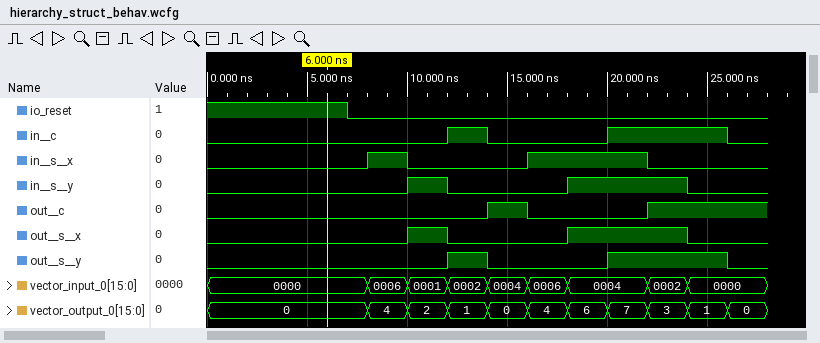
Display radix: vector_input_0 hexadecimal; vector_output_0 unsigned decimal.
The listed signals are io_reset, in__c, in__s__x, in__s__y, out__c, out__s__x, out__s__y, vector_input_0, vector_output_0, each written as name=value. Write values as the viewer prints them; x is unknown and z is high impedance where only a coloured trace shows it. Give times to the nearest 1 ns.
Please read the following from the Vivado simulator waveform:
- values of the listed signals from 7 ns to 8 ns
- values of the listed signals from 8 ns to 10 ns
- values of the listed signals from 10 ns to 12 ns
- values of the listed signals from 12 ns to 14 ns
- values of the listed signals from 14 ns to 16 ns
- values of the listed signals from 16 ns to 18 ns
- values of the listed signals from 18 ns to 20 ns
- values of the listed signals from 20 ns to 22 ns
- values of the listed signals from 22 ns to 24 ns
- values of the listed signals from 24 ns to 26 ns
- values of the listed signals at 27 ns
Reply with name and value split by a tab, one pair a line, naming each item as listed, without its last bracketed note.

values of the listed signals from 7 ns to 8 ns	io_reset=0, in__c=0, in__s__x=0, in__s__y=0, out__c=0, out__s__x=0, out__s__y=0, vector_input_0=0000, vector_output_0=0
values of the listed signals from 8 ns to 10 ns	io_reset=0, in__c=0, in__s__x=1, in__s__y=0, out__c=0, out__s__x=0, out__s__y=0, vector_input_0=0006, vector_output_0=4
values of the listed signals from 10 ns to 12 ns	io_reset=0, in__c=0, in__s__x=0, in__s__y=1, out__c=0, out__s__x=1, out__s__y=0, vector_input_0=0001, vector_output_0=2
values of the listed signals from 12 ns to 14 ns	io_reset=0, in__c=1, in__s__x=0, in__s__y=0, out__c=0, out__s__x=0, out__s__y=1, vector_input_0=0002, vector_output_0=1
values of the listed signals from 14 ns to 16 ns	io_reset=0, in__c=0, in__s__x=0, in__s__y=0, out__c=1, out__s__x=0, out__s__y=0, vector_input_0=0004, vector_output_0=0
values of the listed signals from 16 ns to 18 ns	io_reset=0, in__c=0, in__s__x=1, in__s__y=0, out__c=0, out__s__x=0, out__s__y=0, vector_input_0=0006, vector_output_0=4
values of the listed signals from 18 ns to 20 ns	io_reset=0, in__c=0, in__s__x=1, in__s__y=1, out__c=0, out__s__x=1, out__s__y=0, vector_input_0=0004, vector_output_0=6
values of the listed signals from 20 ns to 22 ns	io_reset=0, in__c=1, in__s__x=1, in__s__y=1, out__c=0, out__s__x=1, out__s__y=1, vector_input_0=0004, vector_output_0=7
values of the listed signals from 22 ns to 24 ns	io_reset=0, in__c=1, in__s__x=0, in__s__y=1, out__c=1, out__s__x=1, out__s__y=1, vector_input_0=0002, vector_output_0=3
values of the listed signals from 24 ns to 26 ns	io_reset=0, in__c=1, in__s__x=0, in__s__y=0, out__c=1, out__s__x=0, out__s__y=1, vector_input_0=0000, vector_output_0=1
values of the listed signals at 27 ns	io_reset=0, in__c=0, in__s__x=0, in__s__y=0, out__c=1, out__s__x=0, out__s__y=0, vector_input_0=0000, vector_output_0=0
